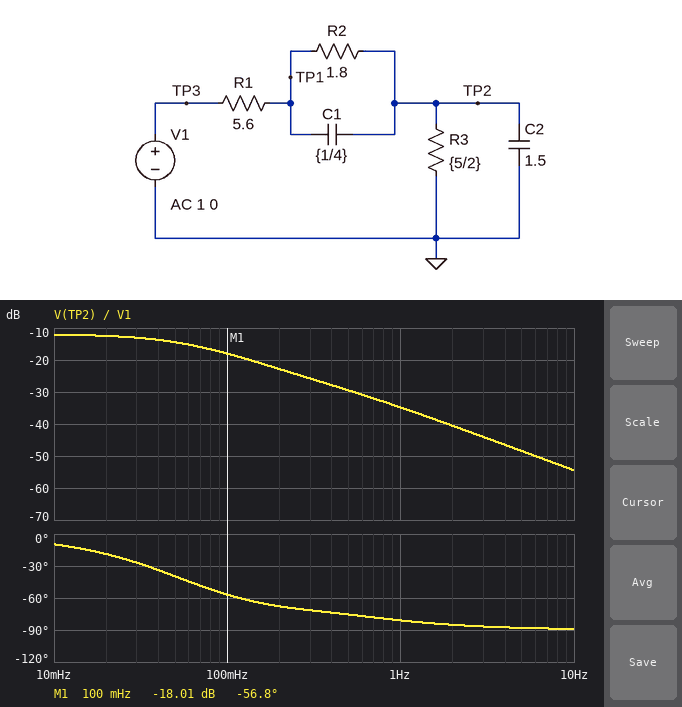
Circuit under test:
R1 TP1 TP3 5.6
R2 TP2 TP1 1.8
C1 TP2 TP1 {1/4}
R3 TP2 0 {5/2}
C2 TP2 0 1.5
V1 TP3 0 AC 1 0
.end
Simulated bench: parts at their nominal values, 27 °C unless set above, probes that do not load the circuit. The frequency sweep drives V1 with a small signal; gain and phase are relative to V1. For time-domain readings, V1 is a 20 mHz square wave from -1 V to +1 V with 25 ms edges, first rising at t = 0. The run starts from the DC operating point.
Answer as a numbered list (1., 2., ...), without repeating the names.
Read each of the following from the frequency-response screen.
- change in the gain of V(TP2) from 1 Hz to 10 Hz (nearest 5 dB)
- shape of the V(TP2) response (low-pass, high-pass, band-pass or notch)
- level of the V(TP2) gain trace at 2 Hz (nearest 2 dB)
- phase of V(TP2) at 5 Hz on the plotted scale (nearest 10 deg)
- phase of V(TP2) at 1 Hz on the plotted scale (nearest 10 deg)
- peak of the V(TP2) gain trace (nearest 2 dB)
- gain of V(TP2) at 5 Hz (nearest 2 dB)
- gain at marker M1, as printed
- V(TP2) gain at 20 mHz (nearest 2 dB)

1. -20 dB
2. low-pass
3. -40 dB
4. -90 deg
5. -80 deg
6. -12 dB
7. -48 dB
8. -18.01 dB
9. -12 dB
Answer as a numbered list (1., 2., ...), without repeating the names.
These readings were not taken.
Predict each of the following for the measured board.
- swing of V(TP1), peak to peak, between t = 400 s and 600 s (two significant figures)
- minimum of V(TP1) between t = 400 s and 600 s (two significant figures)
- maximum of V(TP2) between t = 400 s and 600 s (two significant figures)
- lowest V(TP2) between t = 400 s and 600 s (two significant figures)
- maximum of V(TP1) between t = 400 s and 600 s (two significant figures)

1. 870 mV
2. -430 mV
3. 250 mV
4. -250 mV
5. 430 mV
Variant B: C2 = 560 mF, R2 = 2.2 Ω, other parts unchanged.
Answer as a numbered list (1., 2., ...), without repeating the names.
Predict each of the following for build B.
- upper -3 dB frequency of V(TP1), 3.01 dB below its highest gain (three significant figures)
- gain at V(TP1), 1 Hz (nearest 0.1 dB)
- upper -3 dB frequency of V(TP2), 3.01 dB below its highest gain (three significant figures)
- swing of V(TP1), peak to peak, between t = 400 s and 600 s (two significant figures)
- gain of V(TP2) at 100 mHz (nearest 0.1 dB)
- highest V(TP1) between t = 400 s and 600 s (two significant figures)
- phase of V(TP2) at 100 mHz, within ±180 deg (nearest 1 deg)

1. 311 mHz
2. -16.4 dB
3. 162 mHz
4. 910 mV
5. -13.8 dB
6. 460 mV
7. -29 deg
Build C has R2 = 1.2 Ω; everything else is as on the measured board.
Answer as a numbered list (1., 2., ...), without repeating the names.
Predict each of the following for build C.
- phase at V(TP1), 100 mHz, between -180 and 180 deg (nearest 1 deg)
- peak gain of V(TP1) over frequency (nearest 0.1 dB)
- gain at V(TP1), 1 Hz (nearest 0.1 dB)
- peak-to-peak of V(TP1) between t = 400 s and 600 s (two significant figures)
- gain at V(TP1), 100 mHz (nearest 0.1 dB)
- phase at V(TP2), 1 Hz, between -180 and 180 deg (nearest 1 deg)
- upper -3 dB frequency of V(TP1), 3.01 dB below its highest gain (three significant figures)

1. -27 deg
2. -8.0 dB
3. -19.0 dB
4. 800 mV
5. -11.6 dB
6. -82 deg
7. 82.1 mHz
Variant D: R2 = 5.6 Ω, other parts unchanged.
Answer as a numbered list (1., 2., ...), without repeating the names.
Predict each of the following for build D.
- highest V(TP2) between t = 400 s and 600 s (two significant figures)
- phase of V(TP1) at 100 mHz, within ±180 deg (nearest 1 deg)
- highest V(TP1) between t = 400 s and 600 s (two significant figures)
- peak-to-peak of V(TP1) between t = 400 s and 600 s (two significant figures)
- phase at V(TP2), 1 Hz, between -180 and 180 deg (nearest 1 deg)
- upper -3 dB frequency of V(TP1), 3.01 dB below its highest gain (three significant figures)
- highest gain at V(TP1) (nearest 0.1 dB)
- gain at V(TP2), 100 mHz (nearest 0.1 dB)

1. 180 mV
2. -24 deg
3. 590 mV
4. 1.2 V
5. -80 deg
6. 210 mHz
7. -4.6 dB
8. -20.1 dB
